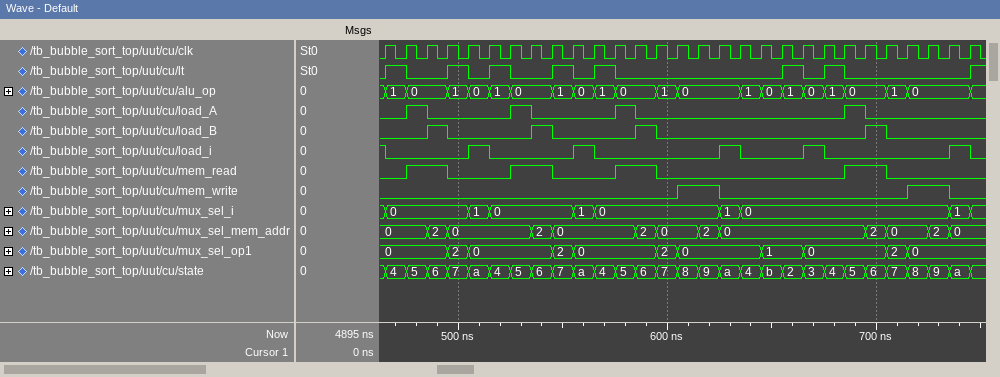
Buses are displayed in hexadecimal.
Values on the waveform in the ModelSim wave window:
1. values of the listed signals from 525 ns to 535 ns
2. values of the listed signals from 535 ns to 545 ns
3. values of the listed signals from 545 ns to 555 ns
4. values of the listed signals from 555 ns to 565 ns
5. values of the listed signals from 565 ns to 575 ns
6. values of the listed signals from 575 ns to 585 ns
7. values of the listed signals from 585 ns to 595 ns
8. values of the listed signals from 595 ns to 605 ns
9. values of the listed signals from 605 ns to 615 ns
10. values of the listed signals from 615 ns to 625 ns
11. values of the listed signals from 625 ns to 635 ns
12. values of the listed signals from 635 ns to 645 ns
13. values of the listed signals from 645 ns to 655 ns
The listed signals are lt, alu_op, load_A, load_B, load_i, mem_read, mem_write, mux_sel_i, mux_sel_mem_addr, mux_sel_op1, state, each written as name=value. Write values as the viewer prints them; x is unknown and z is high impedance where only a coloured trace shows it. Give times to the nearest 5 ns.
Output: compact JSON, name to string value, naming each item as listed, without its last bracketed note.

{"values of the listed signals from 525 ns to 535 ns": "lt=0, alu_op=0, load_A=1, load_B=0, load_i=0, mem_read=1, mem_write=0, mux_sel_i=0, mux_sel_mem_addr=0, mux_sel_op1=0, state=5", "values of the listed signals from 535 ns to 545 ns": "lt=0, alu_op=0, load_A=0, load_B=1, load_i=0, mem_read=1, mem_write=0, mux_sel_i=0, mux_sel_mem_addr=2, mux_sel_op1=0, state=6", "values of the listed signals from 545 ns to 555 ns": "lt=1, alu_op=1, load_A=0, load_B=0, load_i=0, mem_read=0, mem_write=0, mux_sel_i=0, mux_sel_mem_addr=0, mux_sel_op1=2, state=7", "values of the listed signals from 555 ns to 565 ns": "lt=0, alu_op=0, load_A=0, load_B=0, load_i=1, mem_read=0, mem_write=0, mux_sel_i=1, mux_sel_mem_addr=0, mux_sel_op1=0, state=a", "values of the listed signals from 565 ns to 575 ns": "lt=1, alu_op=1, load_A=0, load_B=0, load_i=0, mem_read=0, mem_write=0, mux_sel_i=0, mux_sel_mem_addr=0, mux_sel_op1=0, state=4", "values of the listed signals from 575 ns to 585 ns": "lt=0, alu_op=0, load_A=1, load_B=0, load_i=0, mem_read=1, mem_write=0, mux_sel_i=0, mux_sel_mem_addr=0, mux_sel_op1=0, state=5", "values of the listed signals from 585 ns to 595 ns": "lt=0, alu_op=0, load_A=0, load_B=1, load_i=0, mem_read=1, mem_write=0, mux_sel_i=0, mux_sel_mem_addr=2, mux_sel_op1=0, state=6", "values of the listed signals from 595 ns to 605 ns": "lt=0, alu_op=1, load_A=0, load_B=0, load_i=0, mem_read=0, mem_write=0, mux_sel_i=0, mux_sel_mem_addr=0, mux_sel_op1=2, state=7", "values of the listed signals from 605 ns to 615 ns": "lt=0, alu_op=0, load_A=0, load_B=0, load_i=0, mem_read=0, mem_write=1, mux_sel_i=0, mux_sel_mem_addr=0, mux_sel_op1=0, state=8", "values of the listed signals from 615 ns to 625 ns": "lt=0, alu_op=0, load_A=0, load_B=0, load_i=0, mem_read=0, mem_write=1, mux_sel_i=0, mux_sel_mem_addr=2, mux_sel_op1=0, state=9", "values of the listed signals from 625 ns to 635 ns": "lt=0, alu_op=0, load_A=0, load_B=0, load_i=1, mem_read=0, mem_write=0, mux_sel_i=1, mux_sel_mem_addr=0, mux_sel_op1=0, state=a", "values of the listed signals from 635 ns to 645 ns": "lt=0, alu_op=1, load_A=0, load_B=0, load_i=0, mem_read=0, mem_write=0, mux_sel_i=0, mux_sel_mem_addr=0, mux_sel_op1=0, state=4", "values of the listed signals from 645 ns to 655 ns": "lt=0, alu_op=0, load_A=0, load_B=0, load_i=0, mem_read=0, mem_write=0, mux_sel_i=0, mux_sel_mem_addr=0, mux_sel_op1=1, state=b"}
